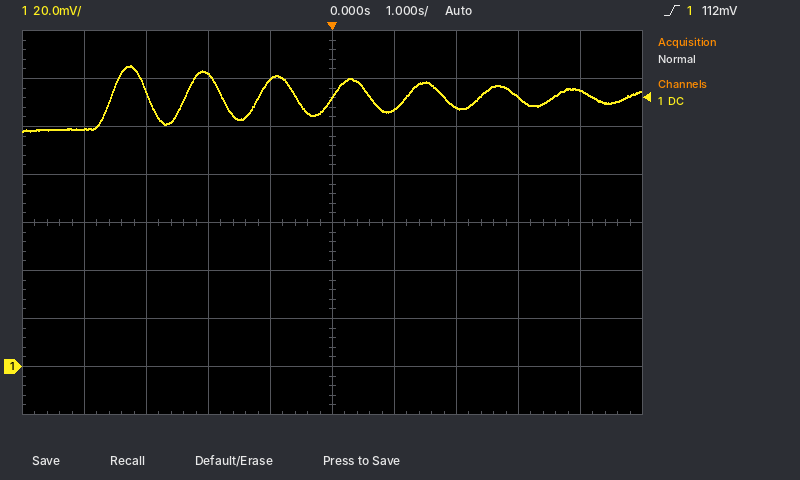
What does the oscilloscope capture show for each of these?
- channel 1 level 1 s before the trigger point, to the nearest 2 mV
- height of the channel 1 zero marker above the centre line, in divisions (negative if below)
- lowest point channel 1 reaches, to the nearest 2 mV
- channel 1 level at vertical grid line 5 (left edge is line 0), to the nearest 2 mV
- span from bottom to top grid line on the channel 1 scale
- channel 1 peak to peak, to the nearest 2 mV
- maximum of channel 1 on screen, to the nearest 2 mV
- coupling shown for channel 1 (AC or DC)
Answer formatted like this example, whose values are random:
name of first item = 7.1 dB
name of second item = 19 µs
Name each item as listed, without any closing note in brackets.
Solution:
channel 1 level 1 s before the trigger point, to the nearest 2 mV = 120 mV
height of the channel 1 zero marker above the centre line, in divisions = -3.0 div
lowest point channel 1 reaches, to the nearest 2 mV = 98 mV
channel 1 level at vertical grid line 5 (left edge is line 0), to the nearest 2 mV = 112 mV
span from bottom to top grid line on the channel 1 scale = 160 mV
channel 1 peak to peak, to the nearest 2 mV = 28 mV
maximum of channel 1 on screen, to the nearest 2 mV = 126 mV
coupling shown for channel 1 = DC
